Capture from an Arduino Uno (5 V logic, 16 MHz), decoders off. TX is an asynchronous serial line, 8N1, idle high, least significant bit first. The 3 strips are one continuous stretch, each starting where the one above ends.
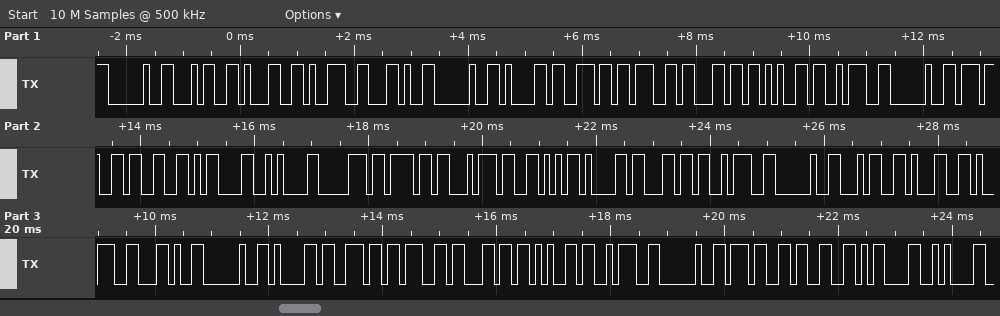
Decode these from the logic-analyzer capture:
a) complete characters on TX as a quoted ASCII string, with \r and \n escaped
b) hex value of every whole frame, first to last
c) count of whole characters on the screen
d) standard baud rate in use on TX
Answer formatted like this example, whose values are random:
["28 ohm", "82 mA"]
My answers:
["\" 419, angle: 73\\r\\npotVal: 419, angle: 73\\r\\n\"", "20 34 31 39 2C 20 61 6E 67 6C 65 3A 20 37 33 0D 0A 70 6F 74 56 61 6C 3A 20 34 31 39 2C 20 61 6E 67 6C 65 3A 20 37 33 0D 0A", "41", "9600 baud"]
